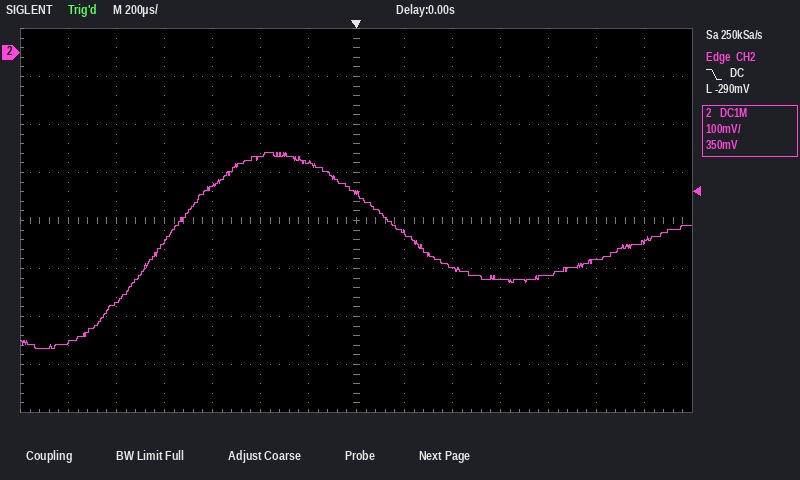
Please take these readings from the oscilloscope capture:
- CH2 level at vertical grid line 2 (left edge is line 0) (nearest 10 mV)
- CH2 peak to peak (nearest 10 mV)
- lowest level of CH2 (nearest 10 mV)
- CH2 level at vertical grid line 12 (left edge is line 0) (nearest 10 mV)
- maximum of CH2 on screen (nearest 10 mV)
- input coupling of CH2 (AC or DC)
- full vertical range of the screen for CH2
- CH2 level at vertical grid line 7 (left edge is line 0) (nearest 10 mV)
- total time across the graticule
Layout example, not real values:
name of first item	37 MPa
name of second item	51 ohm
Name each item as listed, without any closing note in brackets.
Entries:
CH2 level at vertical grid line 2 (left edge is line 0)	-520 mV
CH2 peak to peak	410 mV
lowest level of CH2	-620 mV
CH2 level at vertical grid line 12 (left edge is line 0)	-430 mV
maximum of CH2 on screen	-210 mV
input coupling of CH2	DC
full vertical range of the screen for CH2	800 mV
CH2 level at vertical grid line 7 (left edge is line 0)	-290 mV
total time across the graticule	2.8 ms
